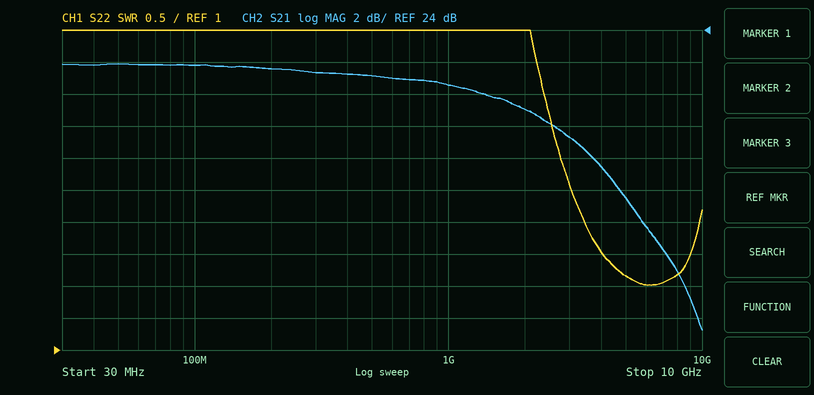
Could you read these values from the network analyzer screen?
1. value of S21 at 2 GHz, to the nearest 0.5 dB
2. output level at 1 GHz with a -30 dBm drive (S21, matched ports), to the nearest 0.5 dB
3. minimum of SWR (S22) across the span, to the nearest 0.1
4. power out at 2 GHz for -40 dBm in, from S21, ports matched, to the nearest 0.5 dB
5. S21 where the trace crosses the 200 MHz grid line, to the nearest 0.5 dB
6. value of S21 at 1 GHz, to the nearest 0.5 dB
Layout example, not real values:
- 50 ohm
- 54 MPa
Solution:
- 19.0 dB
- -9.5 dBm
- 2.0
- -21.0 dBm
- 21.5 dB
- 20.5 dB
